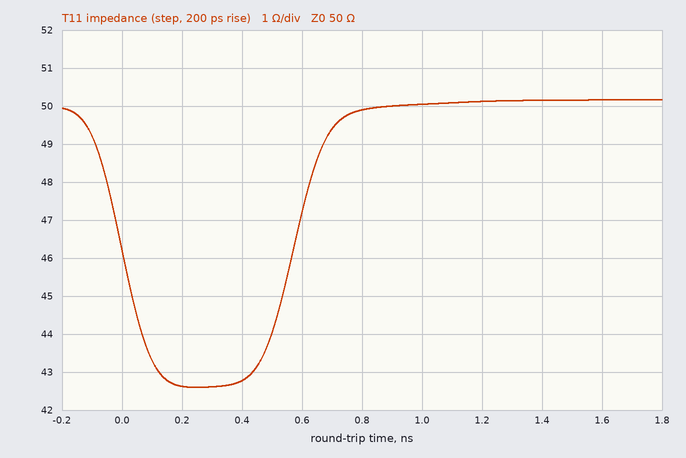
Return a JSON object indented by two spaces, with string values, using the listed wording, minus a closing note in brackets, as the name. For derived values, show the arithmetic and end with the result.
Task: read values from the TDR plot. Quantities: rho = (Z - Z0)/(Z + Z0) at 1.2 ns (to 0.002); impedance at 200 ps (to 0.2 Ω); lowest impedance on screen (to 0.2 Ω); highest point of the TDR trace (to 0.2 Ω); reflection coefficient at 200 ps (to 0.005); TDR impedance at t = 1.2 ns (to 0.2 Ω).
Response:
{
  "rho = (Z - Z0)/(Z + Z0) at 1.2 ns": "(50.2 − 50)/(50.2 + 50) ≈ +0.002",
  "impedance at 200 ps": "42.6 Ω",
  "lowest impedance on screen": "42.6 Ω",
  "highest point of the TDR trace": "50.2 Ω",
  "reflection coefficient at 200 ps": "(42.6 − 50)/(42.6 + 50) ≈ -0.080",
  "TDR impedance at t = 1.2 ns": "50.2 Ω"
}
